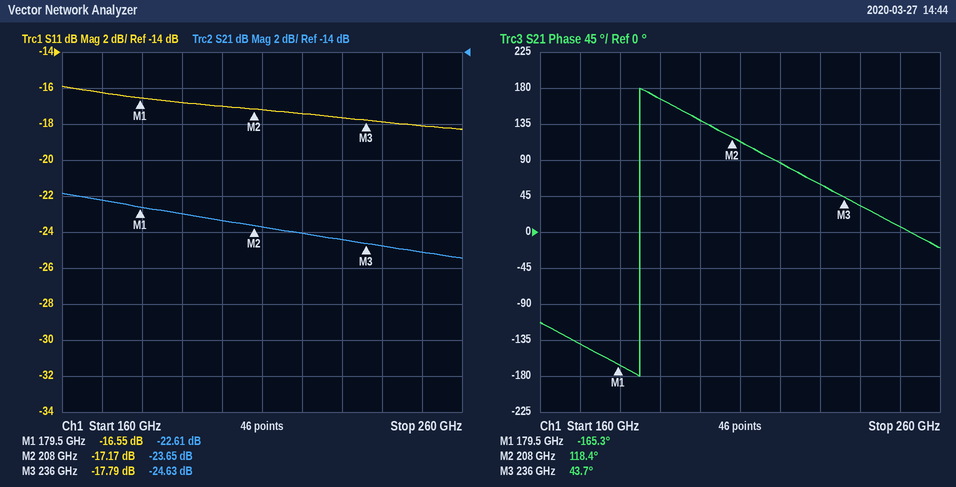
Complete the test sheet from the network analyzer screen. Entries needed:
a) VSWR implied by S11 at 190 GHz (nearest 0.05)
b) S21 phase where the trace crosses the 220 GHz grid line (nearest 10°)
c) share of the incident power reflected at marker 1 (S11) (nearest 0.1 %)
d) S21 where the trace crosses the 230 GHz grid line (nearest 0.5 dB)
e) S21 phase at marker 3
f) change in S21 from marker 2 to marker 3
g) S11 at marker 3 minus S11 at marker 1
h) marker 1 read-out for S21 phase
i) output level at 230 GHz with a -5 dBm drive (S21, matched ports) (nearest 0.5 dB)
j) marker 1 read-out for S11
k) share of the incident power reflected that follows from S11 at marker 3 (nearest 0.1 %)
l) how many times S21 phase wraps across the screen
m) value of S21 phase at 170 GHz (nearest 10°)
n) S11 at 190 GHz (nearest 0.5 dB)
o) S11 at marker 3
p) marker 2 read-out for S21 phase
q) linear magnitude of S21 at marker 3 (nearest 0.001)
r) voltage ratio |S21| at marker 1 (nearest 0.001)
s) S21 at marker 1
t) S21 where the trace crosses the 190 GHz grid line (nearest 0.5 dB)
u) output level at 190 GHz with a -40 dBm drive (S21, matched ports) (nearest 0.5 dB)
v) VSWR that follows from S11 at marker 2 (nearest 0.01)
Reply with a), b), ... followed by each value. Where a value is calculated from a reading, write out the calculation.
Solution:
a) |Γ| = 10^(-17/20) = 0.1413; VSWR = (1 + 0.1413)/(1 − 0.1413) ≈ 1.33, so 1.35 to the nearest 0.05
b) 90°
c) 10^(-16.55/10) ≈ 2.2 %
d) -24.5 dB
e) 43.7°
f) -24.63 − (-23.65) = -0.98 dB
g) -17.79 − (-16.55) = -1.24 dB
h) -165.3°
i) -5 dBm + (-24.5 dB) = -29.5 dBm
j) -16.55 dB
k) 10^(-17.79/10) ≈ 1.7 %
l) 1
m) -140°
n) -17.0 dB
o) -17.79 dB
p) 118.4°
q) 10^(-24.63/20) ≈ 0.059
r) 10^(-22.61/20) ≈ 0.074
s) -22.61 dB
t) -23.0 dB
u) -40 dBm + (-23.0 dB) = -63.0 dBm
v) (1 + 0.1385)/(1 − 0.1385) ≈ 1.32
